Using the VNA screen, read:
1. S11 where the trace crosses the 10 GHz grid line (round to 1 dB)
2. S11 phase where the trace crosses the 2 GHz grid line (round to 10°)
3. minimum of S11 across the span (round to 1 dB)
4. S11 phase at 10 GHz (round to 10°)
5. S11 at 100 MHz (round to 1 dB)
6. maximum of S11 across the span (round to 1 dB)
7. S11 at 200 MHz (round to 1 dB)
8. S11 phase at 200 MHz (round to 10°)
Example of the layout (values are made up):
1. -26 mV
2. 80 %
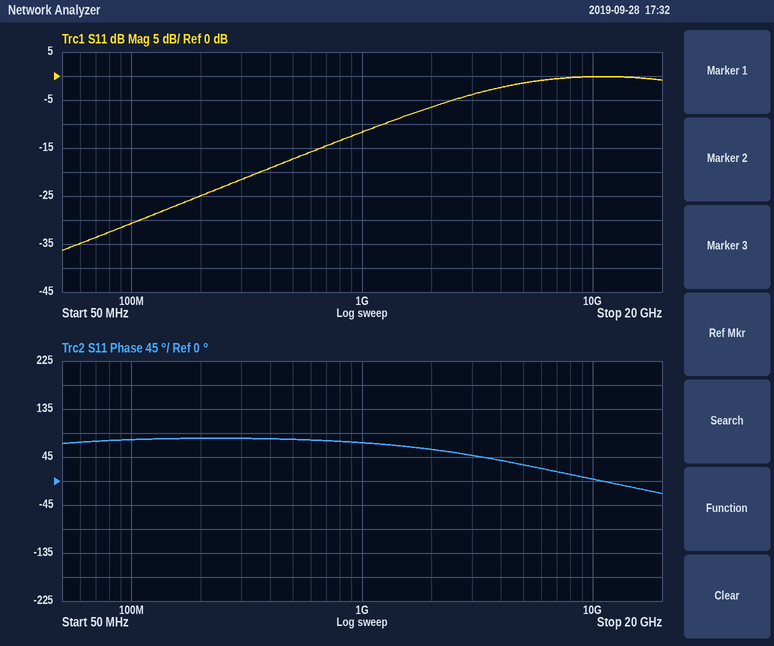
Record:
1. 0 dB
2. 60°
3. -36 dB
4. 0°
5. -31 dB
6. 0 dB
7. -25 dB
8. 80°
